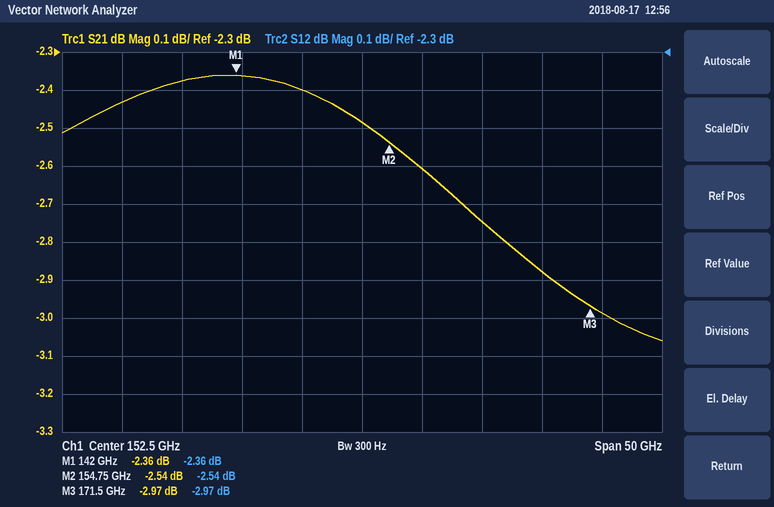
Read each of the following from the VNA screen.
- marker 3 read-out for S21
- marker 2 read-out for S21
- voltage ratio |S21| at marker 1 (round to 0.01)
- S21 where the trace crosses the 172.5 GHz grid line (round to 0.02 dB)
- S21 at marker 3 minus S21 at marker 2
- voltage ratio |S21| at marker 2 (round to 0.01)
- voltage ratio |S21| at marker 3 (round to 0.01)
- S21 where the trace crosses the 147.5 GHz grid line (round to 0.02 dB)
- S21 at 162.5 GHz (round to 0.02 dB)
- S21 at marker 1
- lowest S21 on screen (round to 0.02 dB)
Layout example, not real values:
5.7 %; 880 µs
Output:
-2.97 dB; -2.54 dB; 0.76; -2.98 dB; -0.43 dB; 0.75; 0.71; -2.40 dB; -2.74 dB; -2.36 dB; -3.06 dB
